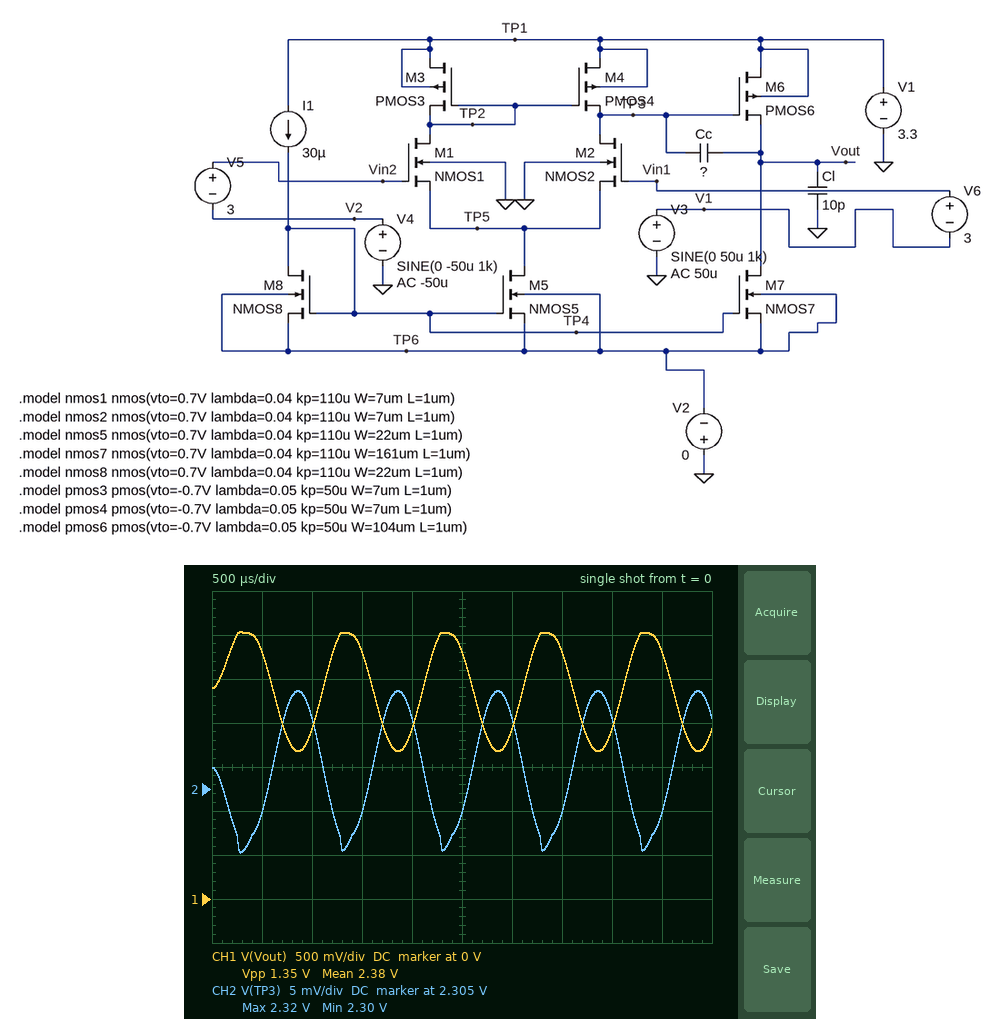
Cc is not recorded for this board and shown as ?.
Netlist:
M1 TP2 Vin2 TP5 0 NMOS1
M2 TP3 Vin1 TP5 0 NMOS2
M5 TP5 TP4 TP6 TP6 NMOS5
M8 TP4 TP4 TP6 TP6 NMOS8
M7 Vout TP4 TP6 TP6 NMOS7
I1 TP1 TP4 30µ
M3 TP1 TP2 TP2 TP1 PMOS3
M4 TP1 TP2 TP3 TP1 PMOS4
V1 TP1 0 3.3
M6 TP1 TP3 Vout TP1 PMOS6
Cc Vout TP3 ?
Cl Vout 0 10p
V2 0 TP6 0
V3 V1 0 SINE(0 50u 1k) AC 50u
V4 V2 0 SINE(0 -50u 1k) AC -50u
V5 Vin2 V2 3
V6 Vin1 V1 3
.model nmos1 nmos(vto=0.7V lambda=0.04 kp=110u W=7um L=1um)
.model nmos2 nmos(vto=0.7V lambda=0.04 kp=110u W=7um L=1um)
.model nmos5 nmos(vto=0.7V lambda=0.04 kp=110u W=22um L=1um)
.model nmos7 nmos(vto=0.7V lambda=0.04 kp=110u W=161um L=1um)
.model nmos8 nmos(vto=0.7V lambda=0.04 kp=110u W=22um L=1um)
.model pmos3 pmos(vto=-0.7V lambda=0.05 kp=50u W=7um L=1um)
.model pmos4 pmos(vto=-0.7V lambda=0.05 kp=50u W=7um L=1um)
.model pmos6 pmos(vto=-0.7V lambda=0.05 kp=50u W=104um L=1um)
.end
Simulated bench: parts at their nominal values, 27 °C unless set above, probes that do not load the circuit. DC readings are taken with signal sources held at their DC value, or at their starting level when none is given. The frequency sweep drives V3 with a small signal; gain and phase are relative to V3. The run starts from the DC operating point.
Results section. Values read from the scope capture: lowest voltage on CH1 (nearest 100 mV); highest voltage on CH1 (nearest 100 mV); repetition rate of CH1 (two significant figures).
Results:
1.7 V
3.0 V
1.0 kHz
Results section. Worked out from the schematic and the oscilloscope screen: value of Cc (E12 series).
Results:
2.2 pF
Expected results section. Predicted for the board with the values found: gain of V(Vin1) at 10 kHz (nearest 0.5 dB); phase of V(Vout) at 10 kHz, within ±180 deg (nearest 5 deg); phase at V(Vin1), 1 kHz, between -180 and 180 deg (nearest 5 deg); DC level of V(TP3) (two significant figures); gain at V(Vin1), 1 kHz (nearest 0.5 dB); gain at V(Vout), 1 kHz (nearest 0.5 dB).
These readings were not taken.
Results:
0 dB
-85 deg
0 deg
2.3 V
0 dB
77.0 dB
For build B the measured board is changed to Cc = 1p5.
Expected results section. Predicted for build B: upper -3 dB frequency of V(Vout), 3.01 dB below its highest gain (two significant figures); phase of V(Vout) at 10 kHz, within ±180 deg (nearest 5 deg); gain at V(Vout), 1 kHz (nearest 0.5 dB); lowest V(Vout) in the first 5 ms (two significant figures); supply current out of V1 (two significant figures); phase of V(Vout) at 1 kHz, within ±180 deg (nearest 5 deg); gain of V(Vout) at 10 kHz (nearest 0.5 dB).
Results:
1.8 kHz
-80 deg
78.0 dB
1.6 V
290 µA
-30 deg
64.0 dB
